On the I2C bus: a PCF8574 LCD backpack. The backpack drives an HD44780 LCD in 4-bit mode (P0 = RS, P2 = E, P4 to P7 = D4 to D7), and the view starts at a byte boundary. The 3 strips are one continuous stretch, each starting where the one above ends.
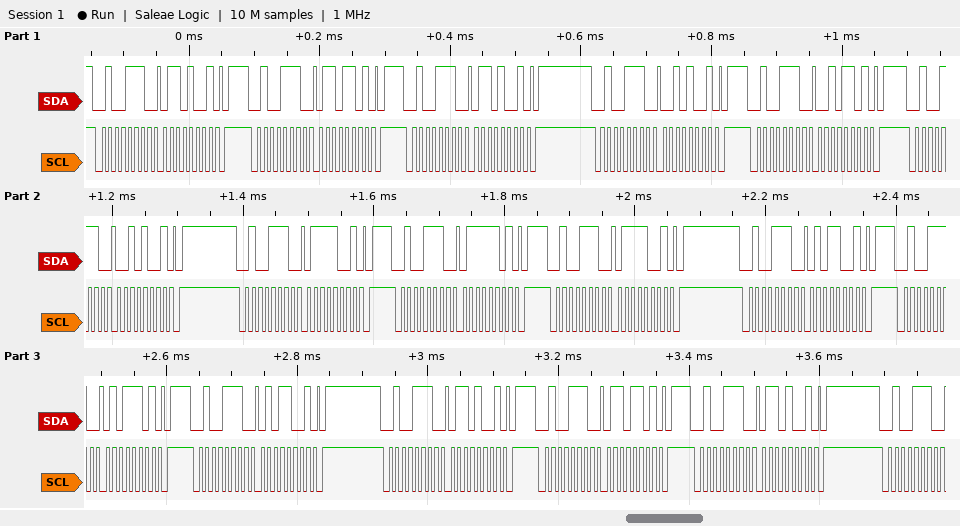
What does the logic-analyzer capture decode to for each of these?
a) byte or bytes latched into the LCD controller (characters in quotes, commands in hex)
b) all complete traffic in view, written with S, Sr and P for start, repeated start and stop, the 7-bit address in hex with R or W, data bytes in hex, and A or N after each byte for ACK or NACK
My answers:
'b' 'u'
S 27W A 69 A P S 27W A 6D A P S 27W A 69 A P S 27W A 29 A P S 27W A 2D A P S 27W A 29 A P S 27W A 79 A P S 27W A 7D A P S 27W A 79 A P S 27W A 59 A P S 27W A 5D A P S 27W A 59 A P S 27W A 69 A P S 27W A 6D A P S 27W A 69 A P S 27W A
